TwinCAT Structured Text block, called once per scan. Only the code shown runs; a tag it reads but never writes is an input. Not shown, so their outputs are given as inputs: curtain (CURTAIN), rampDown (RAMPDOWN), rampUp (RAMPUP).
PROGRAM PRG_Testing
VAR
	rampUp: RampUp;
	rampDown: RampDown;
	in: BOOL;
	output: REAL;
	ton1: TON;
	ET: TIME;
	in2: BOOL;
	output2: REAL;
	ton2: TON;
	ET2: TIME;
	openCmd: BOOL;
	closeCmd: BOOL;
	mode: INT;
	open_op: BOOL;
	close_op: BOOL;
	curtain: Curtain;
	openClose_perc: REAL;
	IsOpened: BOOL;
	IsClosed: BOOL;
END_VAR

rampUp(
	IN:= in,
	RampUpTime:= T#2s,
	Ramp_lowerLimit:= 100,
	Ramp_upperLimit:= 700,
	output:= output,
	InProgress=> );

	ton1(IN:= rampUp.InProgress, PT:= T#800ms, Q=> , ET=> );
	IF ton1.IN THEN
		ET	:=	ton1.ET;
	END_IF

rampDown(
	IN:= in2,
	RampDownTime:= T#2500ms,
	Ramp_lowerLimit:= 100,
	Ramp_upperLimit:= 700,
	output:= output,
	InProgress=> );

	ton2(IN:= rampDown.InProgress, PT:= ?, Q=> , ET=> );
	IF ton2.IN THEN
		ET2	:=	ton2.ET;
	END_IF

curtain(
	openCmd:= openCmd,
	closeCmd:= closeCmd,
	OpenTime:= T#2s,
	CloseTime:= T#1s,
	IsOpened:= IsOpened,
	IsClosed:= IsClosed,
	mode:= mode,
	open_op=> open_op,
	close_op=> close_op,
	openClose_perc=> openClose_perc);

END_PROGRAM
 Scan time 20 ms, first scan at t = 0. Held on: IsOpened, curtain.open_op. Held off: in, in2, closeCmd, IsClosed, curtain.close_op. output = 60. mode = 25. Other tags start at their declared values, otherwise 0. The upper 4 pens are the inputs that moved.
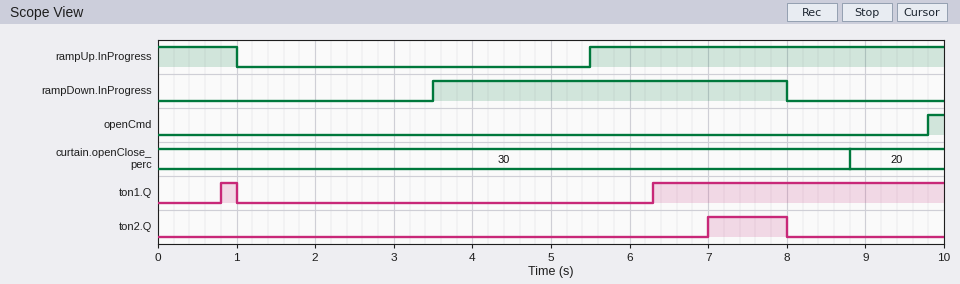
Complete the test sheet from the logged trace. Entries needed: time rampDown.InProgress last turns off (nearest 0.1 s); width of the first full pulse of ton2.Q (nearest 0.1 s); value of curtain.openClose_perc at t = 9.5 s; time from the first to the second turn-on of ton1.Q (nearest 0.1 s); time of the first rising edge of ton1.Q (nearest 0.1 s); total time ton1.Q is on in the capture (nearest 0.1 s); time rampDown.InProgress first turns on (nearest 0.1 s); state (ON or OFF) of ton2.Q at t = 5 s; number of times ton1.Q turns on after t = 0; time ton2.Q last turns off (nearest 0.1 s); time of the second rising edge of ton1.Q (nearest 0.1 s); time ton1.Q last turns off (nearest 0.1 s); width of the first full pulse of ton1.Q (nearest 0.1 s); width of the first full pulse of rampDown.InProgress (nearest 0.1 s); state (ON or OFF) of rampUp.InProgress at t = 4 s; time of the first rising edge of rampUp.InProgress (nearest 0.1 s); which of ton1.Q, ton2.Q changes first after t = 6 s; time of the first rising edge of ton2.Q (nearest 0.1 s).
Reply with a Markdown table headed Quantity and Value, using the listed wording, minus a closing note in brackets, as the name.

| Quantity | Value |
|---|---|
| time rampDown.InProgress last turns off | 8.0 s |
| width of the first full pulse of ton2.Q | 1.0 s |
| value of curtain.openClose_perc at t = 9.5 s | 20 |
| time from the first to the second turn-on of ton1.Q | 5.5 s |
| time of the first rising edge of ton1.Q | 0.8 s |
| total time ton1.Q is on in the capture | 3.9 s |
| time rampDown.InProgress first turns on | 3.5 s |
| state (ON or OFF) of ton2.Q at t = 5 s | OFF |
| number of times ton1.Q turns on after t = 0 | 2 |
| time ton2.Q last turns off | 8.0 s |
| time of the second rising edge of ton1.Q | 6.3 s |
| time ton1.Q last turns off | 1.0 s |
| width of the first full pulse of ton1.Q | 0.2 s |
| width of the first full pulse of rampDown.InProgress | 4.5 s |
| state (ON or OFF) of rampUp.InProgress at t = 4 s | OFF |
| time of the first rising edge of rampUp.InProgress | 5.5 s |
| which of ton1.Q, ton2.Q changes first after t = 6 s | ton1.Q |
| time of the first rising edge of ton2.Q | 7.0 s |
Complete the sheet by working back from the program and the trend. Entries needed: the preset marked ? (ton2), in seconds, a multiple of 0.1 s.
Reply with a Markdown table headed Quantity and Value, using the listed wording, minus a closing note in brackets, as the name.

| Quantity | Value |
|---|---|
| the preset marked ? (ton2), in seconds, a multiple of 0.1 s | 3.5 s |
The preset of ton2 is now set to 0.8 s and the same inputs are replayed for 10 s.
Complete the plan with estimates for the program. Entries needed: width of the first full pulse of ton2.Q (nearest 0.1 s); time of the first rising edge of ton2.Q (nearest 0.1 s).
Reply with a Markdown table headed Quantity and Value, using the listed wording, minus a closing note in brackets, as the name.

| Quantity | Value |
|---|---|
| width of the first full pulse of ton2.Q | 3.7 s |
| time of the first rising edge of ton2.Q | 4.3 s |
